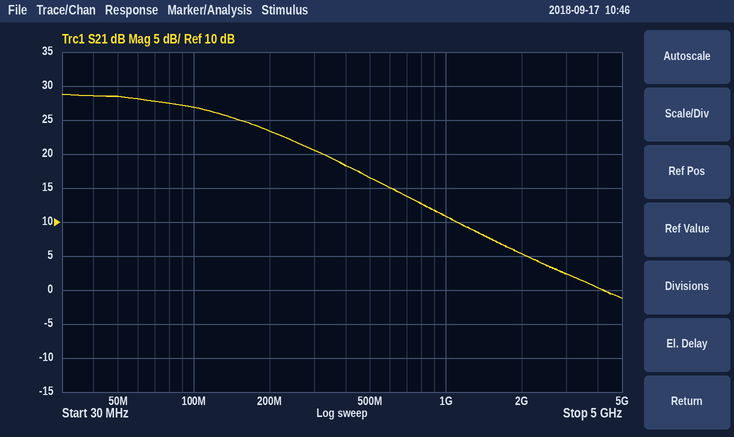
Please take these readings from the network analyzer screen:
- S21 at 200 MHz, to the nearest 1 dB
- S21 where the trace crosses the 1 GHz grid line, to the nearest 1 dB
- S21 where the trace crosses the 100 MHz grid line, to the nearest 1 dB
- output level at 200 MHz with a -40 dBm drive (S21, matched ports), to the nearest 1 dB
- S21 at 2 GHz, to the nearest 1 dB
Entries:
23 dB
11 dB
27 dB
-17 dBm
5 dB
